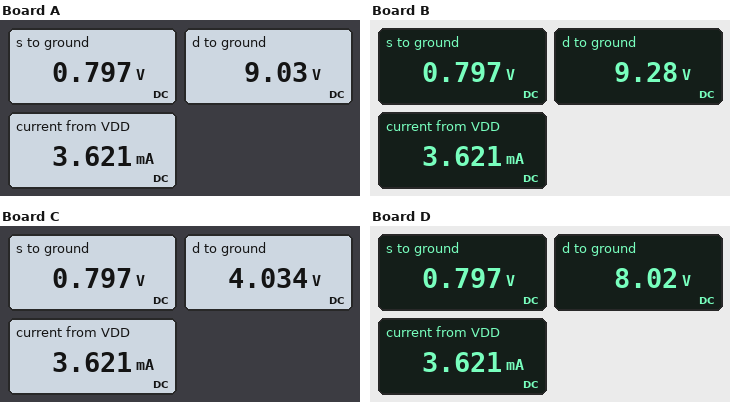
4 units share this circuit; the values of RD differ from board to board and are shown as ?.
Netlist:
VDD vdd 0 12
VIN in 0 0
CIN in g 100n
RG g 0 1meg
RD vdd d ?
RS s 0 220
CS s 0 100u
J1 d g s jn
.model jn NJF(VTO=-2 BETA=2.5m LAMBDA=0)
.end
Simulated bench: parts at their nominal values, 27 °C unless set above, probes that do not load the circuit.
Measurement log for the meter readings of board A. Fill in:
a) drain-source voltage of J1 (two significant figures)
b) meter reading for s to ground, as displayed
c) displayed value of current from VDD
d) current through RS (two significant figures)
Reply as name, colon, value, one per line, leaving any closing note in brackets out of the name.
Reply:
drain-source voltage of J1: 8.2 V
meter reading for s to ground, as displayed: 0.797 V
displayed value of current from VDD: 3.621 mA
current through RS: 3.6 mA
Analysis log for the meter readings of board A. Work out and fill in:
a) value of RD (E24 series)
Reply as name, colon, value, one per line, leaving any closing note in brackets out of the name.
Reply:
value of RD: 820 Ω
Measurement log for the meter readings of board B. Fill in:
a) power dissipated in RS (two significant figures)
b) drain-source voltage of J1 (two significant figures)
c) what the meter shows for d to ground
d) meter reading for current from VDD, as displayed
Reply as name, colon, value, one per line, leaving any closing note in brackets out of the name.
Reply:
power dissipated in RS: 2.9 mW
drain-source voltage of J1: 8.5 V
what the meter shows for d to ground: 9.28 V
meter reading for current from VDD, as displayed: 3.621 mA
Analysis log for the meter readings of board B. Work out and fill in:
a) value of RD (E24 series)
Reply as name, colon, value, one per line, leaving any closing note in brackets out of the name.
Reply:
value of RD: 750 Ω
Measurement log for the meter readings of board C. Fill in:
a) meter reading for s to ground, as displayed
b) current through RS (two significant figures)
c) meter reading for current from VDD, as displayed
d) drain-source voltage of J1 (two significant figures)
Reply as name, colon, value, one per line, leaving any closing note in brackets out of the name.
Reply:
meter reading for s to ground, as displayed: 0.797 V
current through RS: 3.6 mA
meter reading for current from VDD, as displayed: 3.621 mA
drain-source voltage of J1: 3.2 V
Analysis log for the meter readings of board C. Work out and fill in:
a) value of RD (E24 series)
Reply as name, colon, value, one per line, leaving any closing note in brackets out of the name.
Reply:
value of RD: 2.2 kΩ
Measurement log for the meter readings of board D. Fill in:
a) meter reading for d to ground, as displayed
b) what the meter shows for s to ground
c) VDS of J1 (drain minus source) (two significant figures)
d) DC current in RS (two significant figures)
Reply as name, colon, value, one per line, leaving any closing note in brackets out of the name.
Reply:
meter reading for d to ground, as displayed: 8.02 V
what the meter shows for s to ground: 0.797 V
VDS of J1 (drain minus source): 7.2 V
DC current in RS: 3.6 mA
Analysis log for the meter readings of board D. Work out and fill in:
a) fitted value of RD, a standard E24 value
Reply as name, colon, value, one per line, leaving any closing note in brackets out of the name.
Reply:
fitted value of RD, a standard E24 value: 1.1 kΩ
